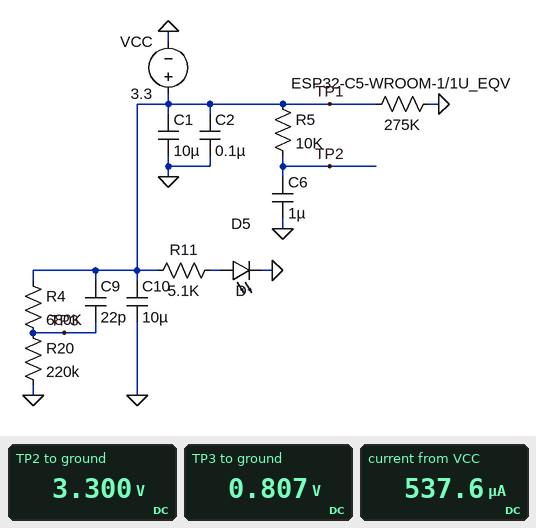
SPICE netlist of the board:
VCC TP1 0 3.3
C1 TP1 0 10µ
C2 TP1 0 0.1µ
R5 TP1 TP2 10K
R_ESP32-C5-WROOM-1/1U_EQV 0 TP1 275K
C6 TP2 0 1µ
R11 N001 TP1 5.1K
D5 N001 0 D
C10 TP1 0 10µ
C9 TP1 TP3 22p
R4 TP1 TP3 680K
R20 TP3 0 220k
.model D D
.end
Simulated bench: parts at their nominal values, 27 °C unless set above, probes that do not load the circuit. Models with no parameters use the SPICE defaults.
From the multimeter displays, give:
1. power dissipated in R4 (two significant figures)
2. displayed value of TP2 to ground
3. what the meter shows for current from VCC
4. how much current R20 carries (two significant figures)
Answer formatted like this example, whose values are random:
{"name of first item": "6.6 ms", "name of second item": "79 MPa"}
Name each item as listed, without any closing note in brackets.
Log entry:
{"power dissipated in R4": "9.1 µW", "displayed value of TP2 to ground": "3.300 V", "what the meter shows for current from VCC": "537.6 µA", "how much current R20 carries": "3.7 µA"}
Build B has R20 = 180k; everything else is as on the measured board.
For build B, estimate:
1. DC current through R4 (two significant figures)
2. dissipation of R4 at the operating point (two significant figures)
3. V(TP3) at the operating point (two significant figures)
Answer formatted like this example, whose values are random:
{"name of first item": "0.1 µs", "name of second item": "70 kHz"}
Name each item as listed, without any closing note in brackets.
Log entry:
{"DC current through R4": "3.8 µA", "dissipation of R4 at the operating point": "10 µW", "V(TP3) at the operating point": "690 mV"}
